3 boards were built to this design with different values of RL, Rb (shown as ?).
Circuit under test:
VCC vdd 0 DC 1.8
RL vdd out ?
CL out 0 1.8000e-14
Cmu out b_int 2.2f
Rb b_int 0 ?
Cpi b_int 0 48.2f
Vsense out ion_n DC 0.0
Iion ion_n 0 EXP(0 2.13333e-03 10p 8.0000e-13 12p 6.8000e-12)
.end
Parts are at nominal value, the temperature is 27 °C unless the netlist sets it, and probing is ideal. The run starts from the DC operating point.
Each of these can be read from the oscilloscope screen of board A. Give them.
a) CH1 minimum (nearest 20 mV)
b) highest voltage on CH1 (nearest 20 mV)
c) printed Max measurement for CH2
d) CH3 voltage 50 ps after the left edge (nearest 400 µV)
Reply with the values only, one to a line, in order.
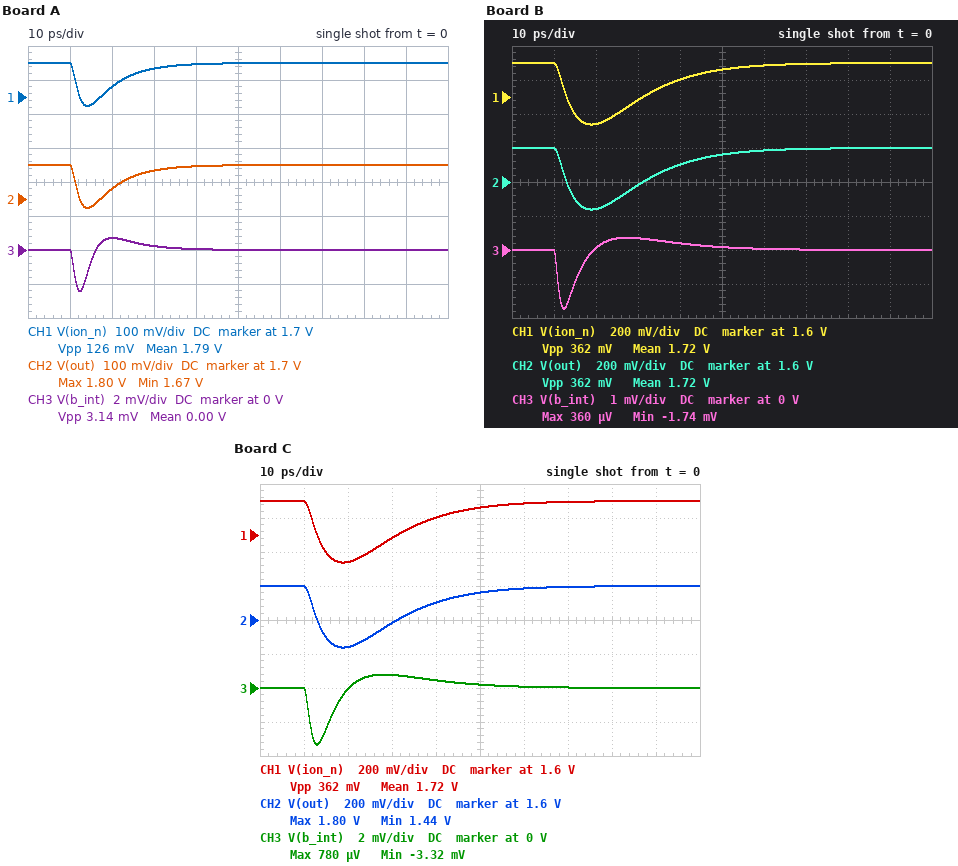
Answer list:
1.68 V
1.80 V
1.80 V
0 V
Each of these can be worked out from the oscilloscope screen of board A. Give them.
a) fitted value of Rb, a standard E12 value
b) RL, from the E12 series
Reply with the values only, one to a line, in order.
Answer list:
33 Ω
82 Ω
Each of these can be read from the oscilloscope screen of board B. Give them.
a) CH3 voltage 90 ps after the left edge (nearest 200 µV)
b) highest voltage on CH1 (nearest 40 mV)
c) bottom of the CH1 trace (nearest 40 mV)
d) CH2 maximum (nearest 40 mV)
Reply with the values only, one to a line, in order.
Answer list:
0 V
1.80 V
1.44 V
1.80 V
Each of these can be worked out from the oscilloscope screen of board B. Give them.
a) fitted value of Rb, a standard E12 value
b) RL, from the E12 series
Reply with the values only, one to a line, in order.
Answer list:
10 Ω
470 Ω
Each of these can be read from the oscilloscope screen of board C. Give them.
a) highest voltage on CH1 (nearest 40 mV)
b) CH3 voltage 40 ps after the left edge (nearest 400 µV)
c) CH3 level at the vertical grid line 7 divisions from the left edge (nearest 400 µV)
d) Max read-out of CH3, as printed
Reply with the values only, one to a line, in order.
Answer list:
1.80 V
400 µV
0 V
780 µV
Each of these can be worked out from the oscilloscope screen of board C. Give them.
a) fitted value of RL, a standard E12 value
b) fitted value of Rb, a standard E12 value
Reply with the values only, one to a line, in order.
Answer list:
470 Ω
22 Ω
